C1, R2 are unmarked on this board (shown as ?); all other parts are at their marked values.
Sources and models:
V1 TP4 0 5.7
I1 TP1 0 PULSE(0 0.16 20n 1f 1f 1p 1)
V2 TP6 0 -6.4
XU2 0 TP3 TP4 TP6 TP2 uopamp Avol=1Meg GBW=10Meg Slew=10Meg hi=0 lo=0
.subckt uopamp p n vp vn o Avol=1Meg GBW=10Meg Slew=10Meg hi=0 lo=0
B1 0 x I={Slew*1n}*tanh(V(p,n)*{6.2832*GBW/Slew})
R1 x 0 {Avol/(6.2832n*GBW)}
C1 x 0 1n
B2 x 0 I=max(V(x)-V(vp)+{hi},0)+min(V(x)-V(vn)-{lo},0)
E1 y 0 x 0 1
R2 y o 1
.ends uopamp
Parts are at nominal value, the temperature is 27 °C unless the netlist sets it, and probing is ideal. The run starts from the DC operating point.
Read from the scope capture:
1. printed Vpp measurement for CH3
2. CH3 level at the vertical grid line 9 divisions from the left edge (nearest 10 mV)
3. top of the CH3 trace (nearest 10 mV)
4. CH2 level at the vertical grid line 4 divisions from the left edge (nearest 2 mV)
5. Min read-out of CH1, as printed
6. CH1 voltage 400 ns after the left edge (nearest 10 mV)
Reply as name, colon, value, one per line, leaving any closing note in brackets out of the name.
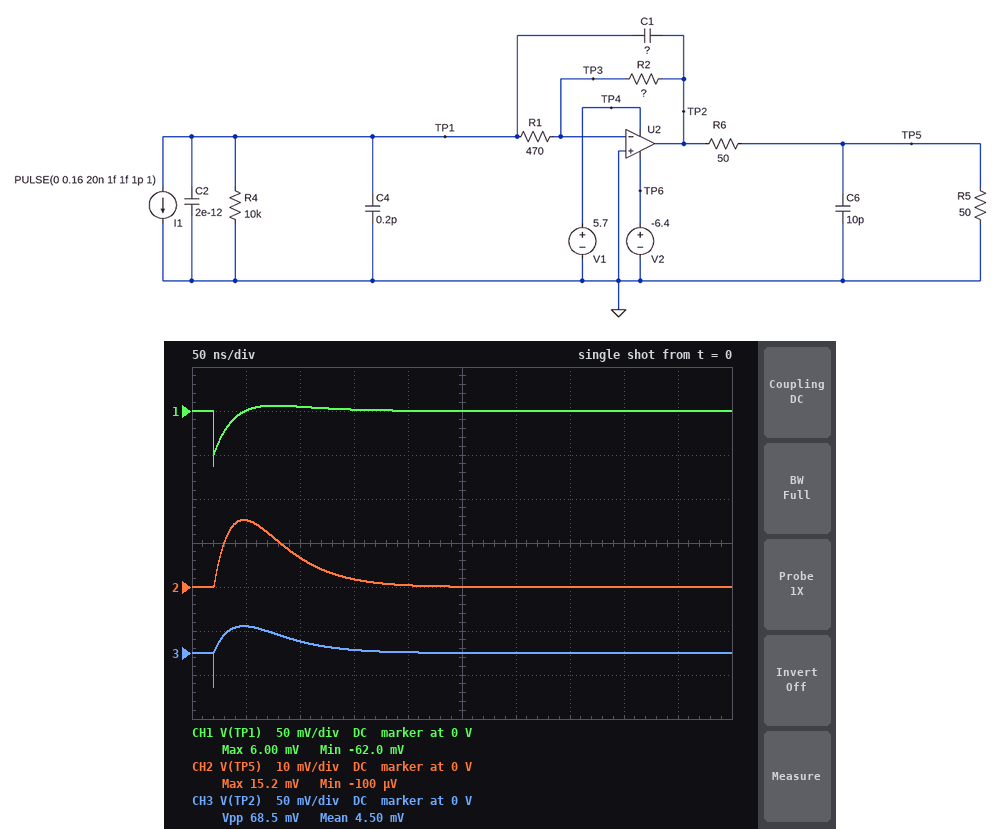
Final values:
printed Vpp measurement for CH3: 68.5 mV
CH3 level at the vertical grid line 9 divisions from the left edge: 0 V
top of the CH3 trace: 30 mV
CH2 level at the vertical grid line 4 divisions from the left edge: 0 V
Min read-out of CH1, as printed: -62.0 mV
CH1 voltage 400 ns after the left edge: 0 V
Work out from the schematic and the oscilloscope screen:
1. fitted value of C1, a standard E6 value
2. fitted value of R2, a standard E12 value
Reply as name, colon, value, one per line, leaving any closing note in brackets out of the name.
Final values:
fitted value of C1, a standard E6 value: 1 pF
fitted value of R2, a standard E12 value: 15 kΩ
